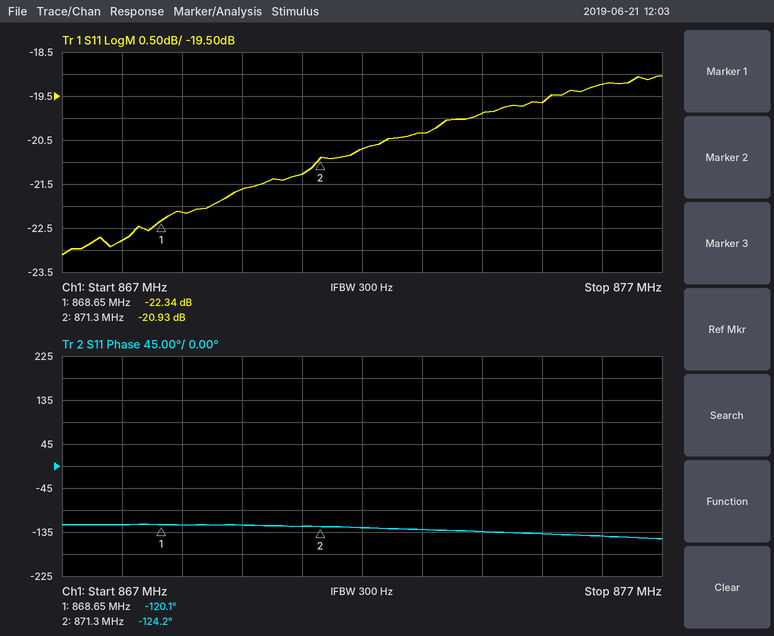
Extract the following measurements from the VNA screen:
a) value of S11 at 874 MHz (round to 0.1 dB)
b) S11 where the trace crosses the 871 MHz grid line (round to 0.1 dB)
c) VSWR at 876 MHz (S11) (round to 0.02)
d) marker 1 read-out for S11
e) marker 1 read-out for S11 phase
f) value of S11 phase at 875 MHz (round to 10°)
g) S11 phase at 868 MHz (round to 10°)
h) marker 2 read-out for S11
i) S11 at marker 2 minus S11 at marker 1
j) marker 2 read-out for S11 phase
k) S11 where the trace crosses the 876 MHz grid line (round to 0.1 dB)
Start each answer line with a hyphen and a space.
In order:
- -19.9 dB
- -21.3 dB
- 1.24
- -22.34 dB
- -120.1°
- -140°
- -120°
- -20.93 dB
- 1.41 dB
- -124.2°
- -19.2 dB
